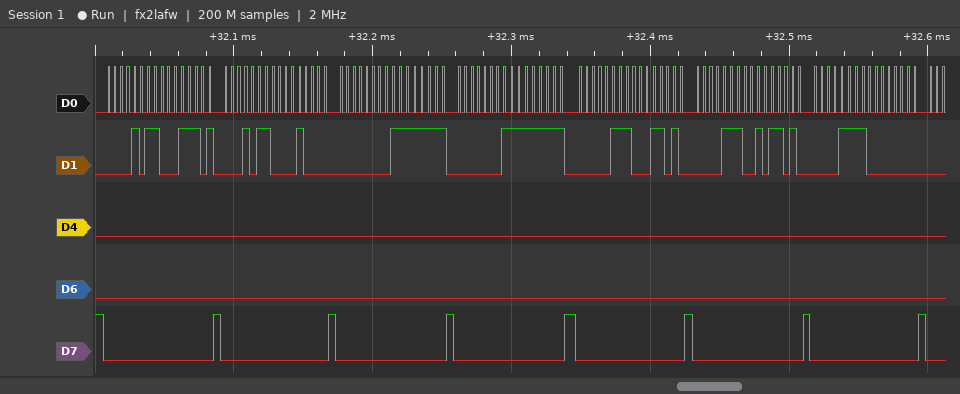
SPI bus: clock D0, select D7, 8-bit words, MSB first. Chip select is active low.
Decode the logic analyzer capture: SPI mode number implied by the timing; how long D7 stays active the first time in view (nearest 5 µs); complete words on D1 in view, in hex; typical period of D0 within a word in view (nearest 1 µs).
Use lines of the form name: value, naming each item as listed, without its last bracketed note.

SPI mode number implied by the timing: 1
how long D7 stays active the first time in view: 80 µs
complete words on D1 in view, in hex: 0B, 1D, 16, 10, 00, FF, 01, FF, 07, 1A, 0E, 5A, 0F, 00
typical period of D0 within a word in view: 5 µs
